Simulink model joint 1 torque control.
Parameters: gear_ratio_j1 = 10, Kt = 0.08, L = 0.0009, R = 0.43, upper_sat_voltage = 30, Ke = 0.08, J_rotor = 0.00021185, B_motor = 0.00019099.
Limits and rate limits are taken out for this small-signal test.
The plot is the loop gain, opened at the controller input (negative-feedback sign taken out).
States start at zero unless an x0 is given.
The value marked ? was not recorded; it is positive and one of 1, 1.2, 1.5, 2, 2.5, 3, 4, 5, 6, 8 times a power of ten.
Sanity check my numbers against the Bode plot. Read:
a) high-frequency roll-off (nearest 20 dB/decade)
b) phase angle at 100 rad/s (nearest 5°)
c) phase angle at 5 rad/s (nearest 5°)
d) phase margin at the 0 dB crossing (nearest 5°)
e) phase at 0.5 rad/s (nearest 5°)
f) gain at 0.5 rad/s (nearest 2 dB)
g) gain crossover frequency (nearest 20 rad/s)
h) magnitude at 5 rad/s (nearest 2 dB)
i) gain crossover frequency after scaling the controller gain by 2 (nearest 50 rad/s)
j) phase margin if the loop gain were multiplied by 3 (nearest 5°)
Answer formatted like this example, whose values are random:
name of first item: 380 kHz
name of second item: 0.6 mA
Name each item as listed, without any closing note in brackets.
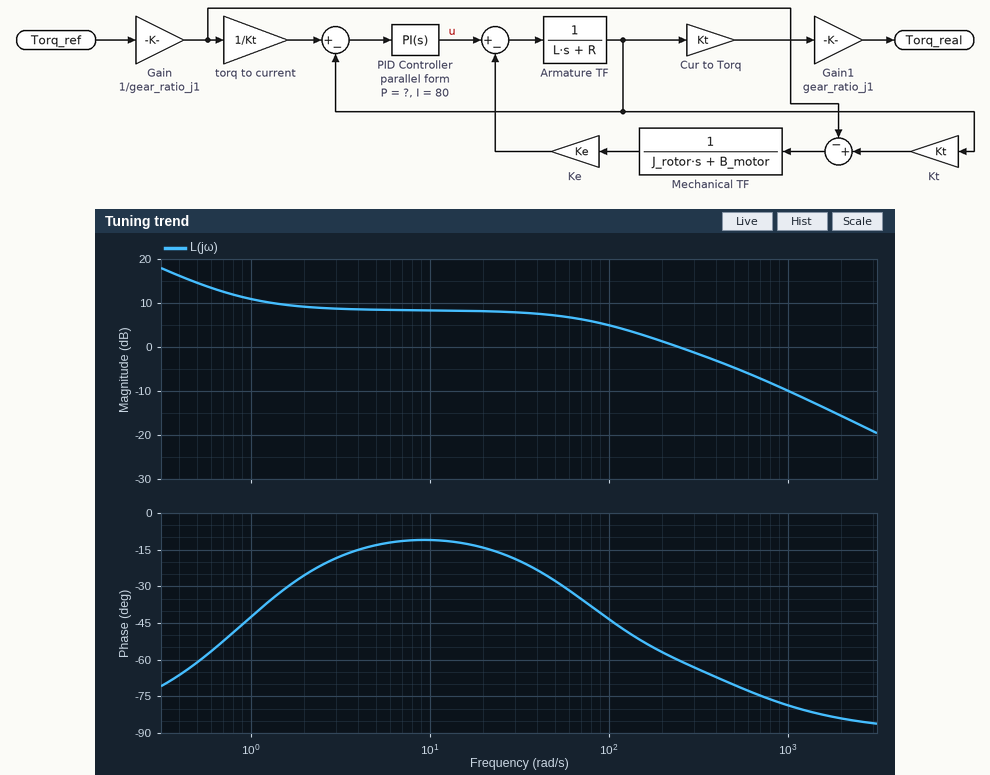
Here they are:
high-frequency roll-off: -20 dB/decade
phase angle at 100 rad/s: -45°
phase angle at 5 rad/s: -15°
phase margin at the 0 dB crossing: 120°
phase at 0.5 rad/s: -60°
gain at 0.5 rad/s: 14 dB
gain crossover frequency: 240 rad/s
magnitude at 5 rad/s: 8 dB
gain crossover frequency after scaling the controller gain by 2: 600 rad/s
phase margin if the loop gain were multiplied by 3: 100°
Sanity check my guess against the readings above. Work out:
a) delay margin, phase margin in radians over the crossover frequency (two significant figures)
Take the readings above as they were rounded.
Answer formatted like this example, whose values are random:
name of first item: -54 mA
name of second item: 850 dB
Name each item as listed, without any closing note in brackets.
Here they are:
delay margin, phase margin in radians over the crossover frequency: 0.0087 s
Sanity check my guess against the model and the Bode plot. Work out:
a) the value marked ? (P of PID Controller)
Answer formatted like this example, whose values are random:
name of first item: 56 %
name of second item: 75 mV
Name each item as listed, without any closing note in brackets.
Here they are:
the value marked ?: 0.3
